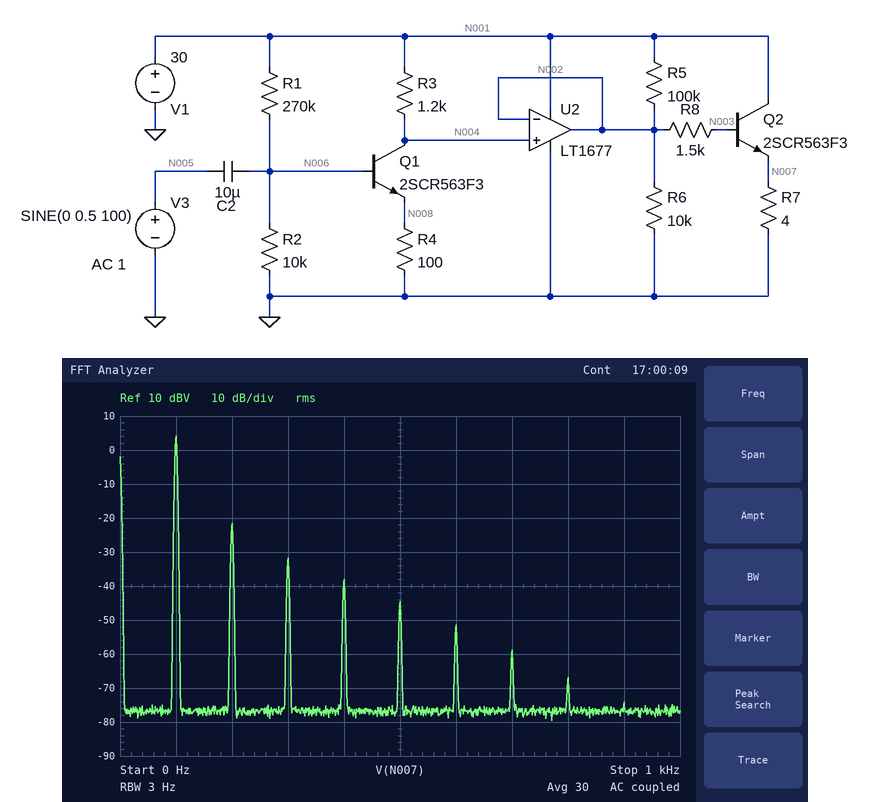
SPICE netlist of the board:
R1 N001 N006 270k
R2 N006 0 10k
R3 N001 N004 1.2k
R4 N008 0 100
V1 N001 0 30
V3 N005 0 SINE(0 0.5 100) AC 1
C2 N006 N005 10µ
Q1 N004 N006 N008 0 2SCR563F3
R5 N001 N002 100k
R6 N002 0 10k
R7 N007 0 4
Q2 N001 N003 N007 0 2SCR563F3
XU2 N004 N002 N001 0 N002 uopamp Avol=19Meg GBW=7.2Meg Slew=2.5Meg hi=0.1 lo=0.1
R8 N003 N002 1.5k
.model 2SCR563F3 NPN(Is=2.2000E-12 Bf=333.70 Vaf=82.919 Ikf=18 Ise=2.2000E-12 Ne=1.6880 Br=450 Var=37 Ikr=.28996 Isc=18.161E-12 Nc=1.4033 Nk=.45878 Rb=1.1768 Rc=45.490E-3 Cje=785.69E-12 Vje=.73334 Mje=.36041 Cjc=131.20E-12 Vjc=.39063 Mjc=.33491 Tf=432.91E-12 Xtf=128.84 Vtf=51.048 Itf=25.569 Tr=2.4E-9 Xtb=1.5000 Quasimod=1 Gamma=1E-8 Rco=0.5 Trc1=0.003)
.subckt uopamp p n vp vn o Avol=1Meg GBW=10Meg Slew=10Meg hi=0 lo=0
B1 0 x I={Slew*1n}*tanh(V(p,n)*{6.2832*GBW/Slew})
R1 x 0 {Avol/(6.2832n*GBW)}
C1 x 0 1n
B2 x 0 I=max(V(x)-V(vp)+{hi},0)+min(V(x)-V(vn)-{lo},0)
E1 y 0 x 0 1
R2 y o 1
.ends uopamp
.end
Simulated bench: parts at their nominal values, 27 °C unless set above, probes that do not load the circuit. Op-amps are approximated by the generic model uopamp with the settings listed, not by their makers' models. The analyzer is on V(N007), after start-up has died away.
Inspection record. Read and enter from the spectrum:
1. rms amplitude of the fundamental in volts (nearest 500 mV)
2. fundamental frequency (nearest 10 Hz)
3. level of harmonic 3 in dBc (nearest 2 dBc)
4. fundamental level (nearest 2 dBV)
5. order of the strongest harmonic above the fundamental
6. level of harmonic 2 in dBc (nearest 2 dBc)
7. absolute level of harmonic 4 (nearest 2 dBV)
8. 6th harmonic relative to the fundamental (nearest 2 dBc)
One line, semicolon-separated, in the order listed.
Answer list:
1.5 V; 100 Hz; -36 dBc; 4 dBV; 2; -26 dBc; -38 dBV; -56 dBc
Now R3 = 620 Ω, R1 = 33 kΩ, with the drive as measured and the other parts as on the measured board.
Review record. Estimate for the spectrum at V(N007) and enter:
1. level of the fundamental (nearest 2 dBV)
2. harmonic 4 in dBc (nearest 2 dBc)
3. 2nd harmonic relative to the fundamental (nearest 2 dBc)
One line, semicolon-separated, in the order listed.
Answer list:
0 dBV; -28 dBc; -20 dBc
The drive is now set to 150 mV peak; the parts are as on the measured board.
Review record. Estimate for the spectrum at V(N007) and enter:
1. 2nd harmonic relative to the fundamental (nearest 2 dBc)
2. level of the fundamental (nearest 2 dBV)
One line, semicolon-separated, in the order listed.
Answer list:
-40 dBc; -6 dBV
